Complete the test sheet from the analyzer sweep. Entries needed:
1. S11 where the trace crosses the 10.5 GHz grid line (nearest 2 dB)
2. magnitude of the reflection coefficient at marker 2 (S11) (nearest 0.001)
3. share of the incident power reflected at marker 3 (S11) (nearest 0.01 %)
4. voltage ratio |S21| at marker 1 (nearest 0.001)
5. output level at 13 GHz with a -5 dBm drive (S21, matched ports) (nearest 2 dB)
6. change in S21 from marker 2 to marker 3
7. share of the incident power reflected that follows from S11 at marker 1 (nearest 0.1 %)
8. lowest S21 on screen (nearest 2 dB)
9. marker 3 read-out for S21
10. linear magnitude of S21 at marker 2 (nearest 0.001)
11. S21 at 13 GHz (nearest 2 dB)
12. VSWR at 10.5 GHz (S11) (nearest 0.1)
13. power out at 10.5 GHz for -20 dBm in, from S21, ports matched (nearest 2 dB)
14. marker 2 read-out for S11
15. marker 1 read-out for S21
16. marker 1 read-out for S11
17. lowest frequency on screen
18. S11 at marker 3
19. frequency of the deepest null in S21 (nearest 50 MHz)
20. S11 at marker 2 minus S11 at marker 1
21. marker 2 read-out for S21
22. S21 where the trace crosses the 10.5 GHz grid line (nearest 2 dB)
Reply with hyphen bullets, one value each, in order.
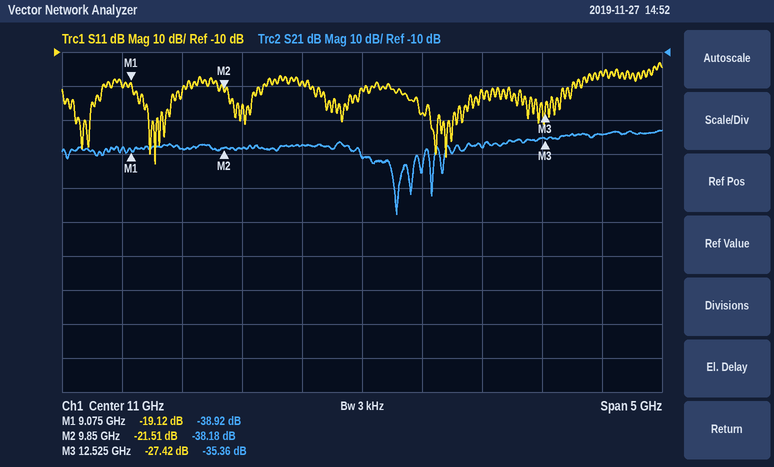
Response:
- -18 dB
- 0.084
- 0.18 %
- 0.011
- -40 dBm
- 2.82 dB
- 1.2 %
- -58 dB
- -35.36 dB
- 0.012
- -34 dB
- 1.3
- -58 dBm
- -21.51 dB
- -38.92 dB
- -19.12 dB
- 8.5 GHz
- -27.42 dB
- 11.30 GHz
- -2.39 dB
- -38.18 dB
- -38 dB
